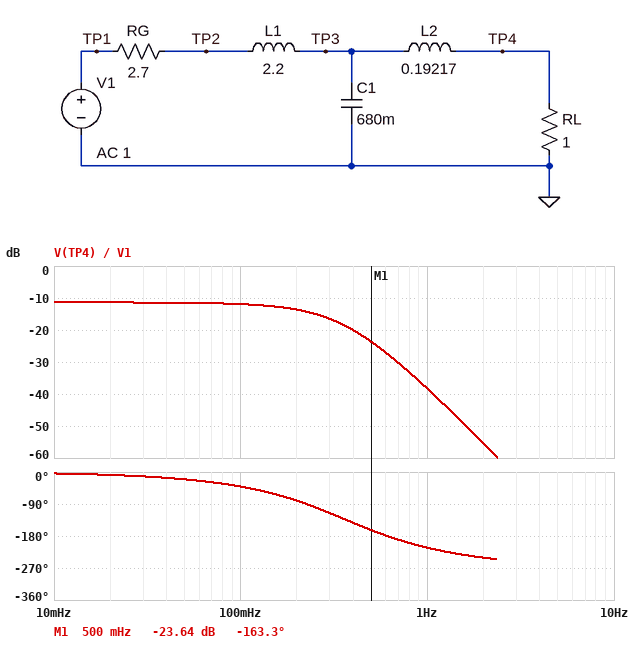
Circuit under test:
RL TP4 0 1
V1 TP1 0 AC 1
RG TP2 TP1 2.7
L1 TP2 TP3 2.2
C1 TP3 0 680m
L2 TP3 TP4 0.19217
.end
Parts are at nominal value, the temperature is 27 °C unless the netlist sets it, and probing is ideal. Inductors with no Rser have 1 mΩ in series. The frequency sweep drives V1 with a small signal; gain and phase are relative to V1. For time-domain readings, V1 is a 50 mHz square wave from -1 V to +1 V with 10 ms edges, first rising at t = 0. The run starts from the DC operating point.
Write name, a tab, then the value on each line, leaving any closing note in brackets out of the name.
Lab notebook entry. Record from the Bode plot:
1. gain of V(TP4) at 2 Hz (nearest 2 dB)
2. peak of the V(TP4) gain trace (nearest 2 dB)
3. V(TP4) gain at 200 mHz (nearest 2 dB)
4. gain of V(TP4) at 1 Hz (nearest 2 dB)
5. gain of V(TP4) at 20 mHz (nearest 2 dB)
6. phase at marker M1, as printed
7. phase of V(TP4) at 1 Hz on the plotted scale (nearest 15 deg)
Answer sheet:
gain of V(TP4) at 2 Hz	-56 dB
peak of the V(TP4) gain trace	-12 dB
V(TP4) gain at 200 mHz	-14 dB
gain of V(TP4) at 1 Hz	-38 dB
gain of V(TP4) at 20 mHz	-12 dB
phase at marker M1, as printed	-163.3 deg
phase of V(TP4) at 1 Hz on the plotted scale	-210 deg
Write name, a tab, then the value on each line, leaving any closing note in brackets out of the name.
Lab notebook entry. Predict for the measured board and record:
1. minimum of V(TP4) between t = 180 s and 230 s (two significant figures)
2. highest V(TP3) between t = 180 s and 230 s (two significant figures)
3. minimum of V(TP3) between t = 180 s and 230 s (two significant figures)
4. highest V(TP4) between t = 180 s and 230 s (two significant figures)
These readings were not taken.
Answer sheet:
minimum of V(TP4) between t = 180 s and 230 s	-270 mV
highest V(TP3) between t = 180 s and 230 s	270 mV
minimum of V(TP3) between t = 180 s and 230 s	-270 mV
highest V(TP4) between t = 180 s and 230 s	270 mV
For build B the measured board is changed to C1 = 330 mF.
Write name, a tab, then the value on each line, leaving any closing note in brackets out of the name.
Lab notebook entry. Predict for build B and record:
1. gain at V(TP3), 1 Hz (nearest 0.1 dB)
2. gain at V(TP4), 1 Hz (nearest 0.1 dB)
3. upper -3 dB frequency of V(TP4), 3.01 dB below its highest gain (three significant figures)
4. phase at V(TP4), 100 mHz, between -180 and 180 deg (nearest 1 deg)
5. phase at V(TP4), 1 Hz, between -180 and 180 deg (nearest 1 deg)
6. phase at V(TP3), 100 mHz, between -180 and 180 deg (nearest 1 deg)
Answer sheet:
gain at V(TP3), 1 Hz	-26.9 dB
gain at V(TP4), 1 Hz	-30.8 dB
upper -3 dB frequency of V(TP4), 3.01 dB below its highest gain	295 mHz
phase at V(TP4), 100 mHz, between -180 and 180 deg	-31 deg
phase at V(TP4), 1 Hz, between -180 and 180 deg	156 deg
phase at V(TP3), 100 mHz, between -180 and 180 deg	-24 deg
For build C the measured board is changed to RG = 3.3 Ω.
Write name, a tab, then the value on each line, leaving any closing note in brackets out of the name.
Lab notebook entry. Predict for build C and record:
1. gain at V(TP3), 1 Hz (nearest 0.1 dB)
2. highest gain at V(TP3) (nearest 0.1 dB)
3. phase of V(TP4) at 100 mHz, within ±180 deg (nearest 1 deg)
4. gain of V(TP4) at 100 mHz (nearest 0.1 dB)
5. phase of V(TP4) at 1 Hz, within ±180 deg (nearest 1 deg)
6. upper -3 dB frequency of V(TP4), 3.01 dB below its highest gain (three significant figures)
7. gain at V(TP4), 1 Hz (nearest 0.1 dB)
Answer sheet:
gain at V(TP3), 1 Hz	-34.5 dB
highest gain at V(TP3)	-12.7 dB
phase of V(TP4) at 100 mHz, within ±180 deg	-39 deg
gain of V(TP4) at 100 mHz	-13.1 dB
phase of V(TP4) at 1 Hz, within ±180 deg	150 deg
upper -3 dB frequency of V(TP4), 3.01 dB below its highest gain	244 mHz
gain at V(TP4), 1 Hz	-38.4 dB
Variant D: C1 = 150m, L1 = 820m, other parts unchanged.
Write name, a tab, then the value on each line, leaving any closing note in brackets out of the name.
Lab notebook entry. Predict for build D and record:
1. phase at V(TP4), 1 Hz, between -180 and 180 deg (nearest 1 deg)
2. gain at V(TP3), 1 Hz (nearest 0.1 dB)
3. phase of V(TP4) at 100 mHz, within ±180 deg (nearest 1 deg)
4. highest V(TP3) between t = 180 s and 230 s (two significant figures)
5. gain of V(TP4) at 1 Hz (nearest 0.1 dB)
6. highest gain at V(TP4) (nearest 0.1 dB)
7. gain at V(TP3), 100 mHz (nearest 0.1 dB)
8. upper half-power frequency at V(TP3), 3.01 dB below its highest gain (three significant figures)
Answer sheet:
phase at V(TP4), 1 Hz, between -180 and 180 deg	-144 deg
gain at V(TP3), 1 Hz	-10.4 dB
phase of V(TP4) at 100 mHz, within ±180 deg	-14 deg
highest V(TP3) between t = 180 s and 230 s	360 mV
gain of V(TP4) at 1 Hz	-14.3 dB
highest gain at V(TP4)	-11.4 dB
gain at V(TP3), 100 mHz	-11.4 dB
upper half-power frequency at V(TP3), 3.01 dB below its highest gain	1.20 Hz
